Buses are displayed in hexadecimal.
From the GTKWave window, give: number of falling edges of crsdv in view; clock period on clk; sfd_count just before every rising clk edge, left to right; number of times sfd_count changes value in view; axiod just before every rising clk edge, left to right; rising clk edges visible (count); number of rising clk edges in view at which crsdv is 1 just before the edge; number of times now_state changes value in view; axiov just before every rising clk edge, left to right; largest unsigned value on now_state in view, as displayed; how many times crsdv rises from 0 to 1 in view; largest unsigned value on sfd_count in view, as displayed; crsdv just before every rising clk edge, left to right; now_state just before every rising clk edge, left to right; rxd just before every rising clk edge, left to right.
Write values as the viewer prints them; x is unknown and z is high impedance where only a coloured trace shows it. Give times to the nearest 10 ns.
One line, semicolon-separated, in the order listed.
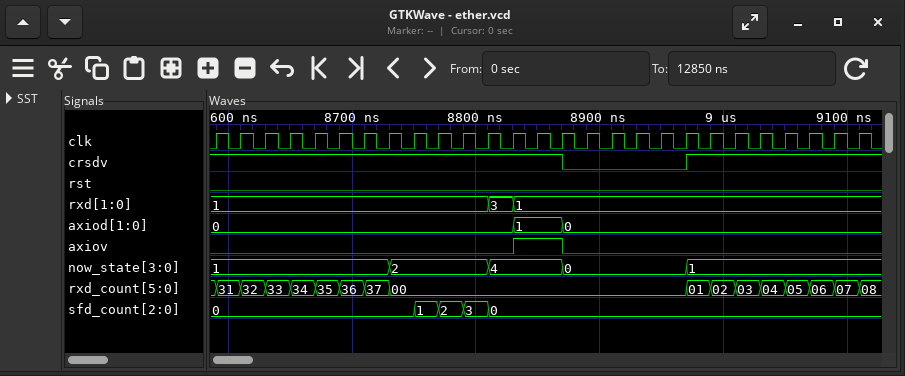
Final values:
1; 20 ns; 0, 0, 0, 0, 0, 0, 0, 0, 0, 1, 2, 3, 0, 0, 0, 0, 0, 0, 0, 0, 0, 0, 0, 0, 0, 0, 0; 4; 0, 0, 0, 0, 0, 0, 0, 0, 0, 0, 0, 0, 0, 1, 1, 0, 0, 0, 0, 0, 0, 0, 0, 0, 0, 0, 0; 27; 22; 4; 0 0 0 0 0 0 0 0 0 0 0 0 0 1 1 0 0 0 0 0 0 0 0 0 0 0 0; 4; 1; 3; 1 1 1 1 1 1 1 1 1 1 1 1 1 1 1 0 0 0 0 0 1 1 1 1 1 1 1; 1, 1, 1, 1, 1, 1, 1, 1, 2, 2, 2, 2, 4, 4, 4, 0, 0, 0, 0, 0, 1, 1, 1, 1, 1, 1, 1; 1, 1, 1, 1, 1, 1, 1, 1, 1, 1, 1, 1, 3, 1, 1, 1, 1, 1, 1, 1, 1, 1, 1, 1, 1, 1, 1
